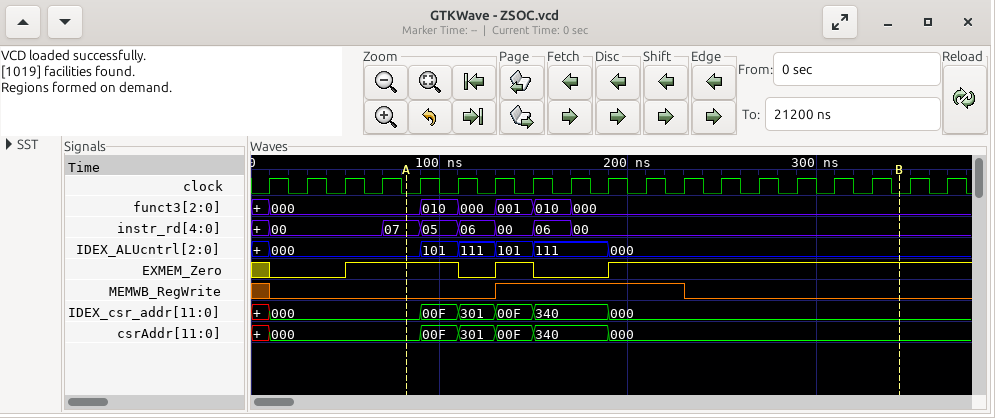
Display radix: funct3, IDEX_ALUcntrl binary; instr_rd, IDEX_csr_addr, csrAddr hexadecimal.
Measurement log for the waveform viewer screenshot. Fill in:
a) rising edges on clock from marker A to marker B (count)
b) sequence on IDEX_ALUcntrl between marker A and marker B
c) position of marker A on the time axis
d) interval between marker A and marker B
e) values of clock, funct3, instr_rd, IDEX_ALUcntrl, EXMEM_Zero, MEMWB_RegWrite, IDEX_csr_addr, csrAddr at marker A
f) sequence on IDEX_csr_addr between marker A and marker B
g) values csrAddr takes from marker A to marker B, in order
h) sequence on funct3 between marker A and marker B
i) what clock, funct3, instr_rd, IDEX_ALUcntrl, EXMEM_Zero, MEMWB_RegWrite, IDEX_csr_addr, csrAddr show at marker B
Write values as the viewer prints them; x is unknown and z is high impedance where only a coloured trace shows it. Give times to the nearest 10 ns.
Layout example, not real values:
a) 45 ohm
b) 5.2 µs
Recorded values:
a) 13
b) 000, 101, 111, 101, 111, 000
c) 80 ns
d) 260 ns
e) clock=0, funct3=000, instr_rd=07, IDEX_ALUcntrl=000, EXMEM_Zero=1, MEMWB_RegWrite=0, IDEX_csr_addr=000, csrAddr=000
f) 000, 00F, 301, 00F, 340, 000
g) 000, 00F, 301, 00F, 340, 000
h) 000, 010, 000, 001, 010, 000
i) clock=0, funct3=000, instr_rd=00, IDEX_ALUcntrl=000, EXMEM_Zero=1, MEMWB_RegWrite=0, IDEX_csr_addr=000, csrAddr=000
